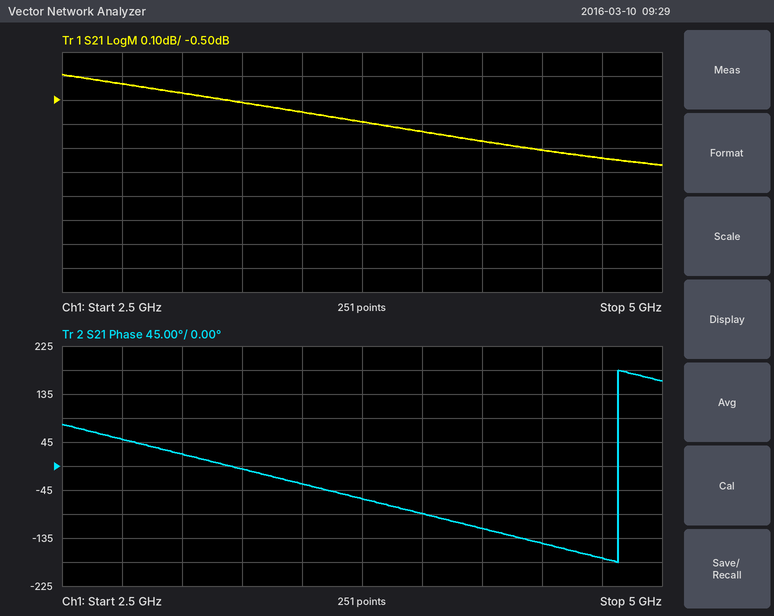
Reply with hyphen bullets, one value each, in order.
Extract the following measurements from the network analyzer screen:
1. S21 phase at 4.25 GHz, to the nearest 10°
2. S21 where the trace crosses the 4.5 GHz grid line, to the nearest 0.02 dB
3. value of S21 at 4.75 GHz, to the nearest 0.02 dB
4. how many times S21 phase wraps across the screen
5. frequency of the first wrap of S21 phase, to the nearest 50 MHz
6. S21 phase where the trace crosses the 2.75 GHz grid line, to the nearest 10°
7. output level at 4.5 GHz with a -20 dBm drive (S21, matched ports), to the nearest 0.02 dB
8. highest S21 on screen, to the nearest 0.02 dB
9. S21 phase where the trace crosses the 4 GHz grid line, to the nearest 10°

- -120°
- -0.70 dB
- -0.74 dB
- 1
- 4.80 GHz
- 50°
- -20.70 dBm
- -0.40 dB
- -90°
